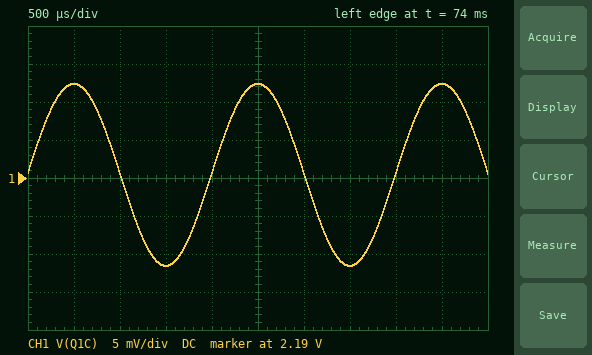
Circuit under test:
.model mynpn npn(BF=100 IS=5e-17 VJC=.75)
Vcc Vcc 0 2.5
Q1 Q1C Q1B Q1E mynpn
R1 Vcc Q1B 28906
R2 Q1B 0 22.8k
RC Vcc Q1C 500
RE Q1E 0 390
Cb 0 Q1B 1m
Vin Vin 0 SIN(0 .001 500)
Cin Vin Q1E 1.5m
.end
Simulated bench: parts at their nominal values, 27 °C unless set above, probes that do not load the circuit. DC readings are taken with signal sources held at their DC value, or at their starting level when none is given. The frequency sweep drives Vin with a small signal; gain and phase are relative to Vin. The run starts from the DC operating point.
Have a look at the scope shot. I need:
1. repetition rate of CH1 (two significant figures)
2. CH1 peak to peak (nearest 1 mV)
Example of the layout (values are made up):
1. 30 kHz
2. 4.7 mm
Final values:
1. 500 Hz
2. 24 mV
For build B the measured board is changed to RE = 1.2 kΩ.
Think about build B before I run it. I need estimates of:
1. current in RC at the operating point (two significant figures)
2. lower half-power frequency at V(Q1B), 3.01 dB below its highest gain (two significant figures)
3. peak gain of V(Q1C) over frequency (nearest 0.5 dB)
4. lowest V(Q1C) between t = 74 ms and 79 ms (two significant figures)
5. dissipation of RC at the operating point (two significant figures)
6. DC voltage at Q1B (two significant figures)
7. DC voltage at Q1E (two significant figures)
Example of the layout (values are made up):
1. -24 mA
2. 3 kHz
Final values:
1. 260 µA
2. 13 mHz
3. 14.0 dB
4. 2.4 V
5. 33 µW
6. 1.1 V
7. 310 mV
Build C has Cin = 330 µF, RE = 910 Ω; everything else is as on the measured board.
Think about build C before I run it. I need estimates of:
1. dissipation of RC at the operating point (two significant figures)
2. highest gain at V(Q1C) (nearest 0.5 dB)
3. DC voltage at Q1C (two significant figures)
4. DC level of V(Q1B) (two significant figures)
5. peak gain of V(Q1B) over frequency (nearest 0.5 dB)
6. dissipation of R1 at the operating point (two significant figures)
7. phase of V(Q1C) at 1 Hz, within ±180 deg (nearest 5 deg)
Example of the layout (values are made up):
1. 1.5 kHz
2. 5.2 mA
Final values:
1. 53 µW
2. 16.0 dB
3. 2.3 V
4. 1.1 V
5. -50.5 dB
6. 72 µW
7. 80 deg
